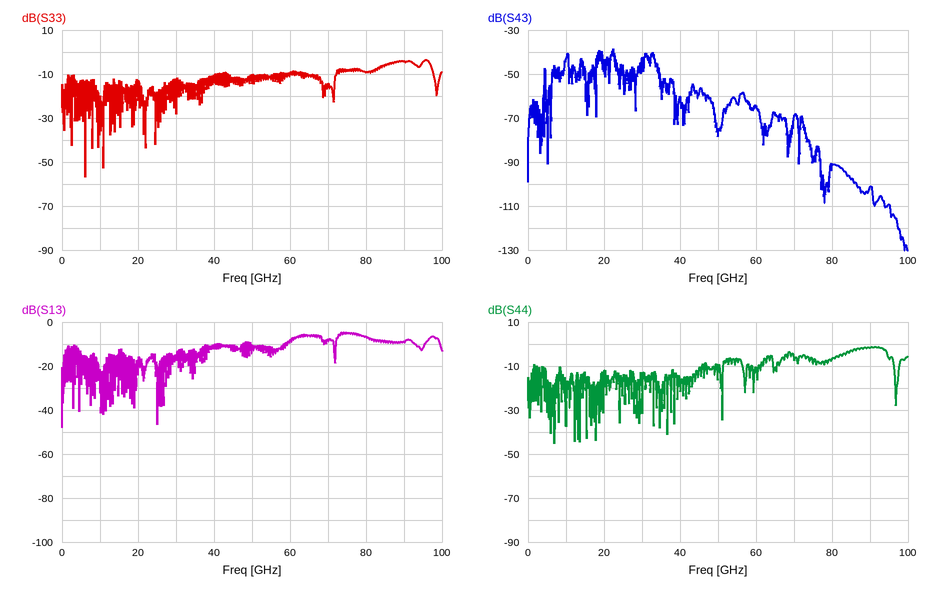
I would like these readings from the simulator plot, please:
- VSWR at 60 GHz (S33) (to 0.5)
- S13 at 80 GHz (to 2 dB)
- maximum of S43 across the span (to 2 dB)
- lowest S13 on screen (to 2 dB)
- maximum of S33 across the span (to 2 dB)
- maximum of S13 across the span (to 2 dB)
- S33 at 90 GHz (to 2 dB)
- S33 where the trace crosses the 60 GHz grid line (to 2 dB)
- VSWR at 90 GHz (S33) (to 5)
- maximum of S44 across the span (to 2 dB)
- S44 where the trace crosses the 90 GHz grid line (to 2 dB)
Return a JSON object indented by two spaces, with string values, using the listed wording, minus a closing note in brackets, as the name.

{
  "VSWR at 60 GHz (S33)": "2.0",
  "S13 at 80 GHz": "-6 dB",
  "maximum of S43 across the span": "-38 dB",
  "lowest S13 on screen": "-48 dB",
  "maximum of S33 across the span": "-4 dB",
  "maximum of S13 across the span": "-4 dB",
  "S33 at 90 GHz": "-4 dB",
  "S33 where the trace crosses the 60 GHz grid line": "-10 dB",
  "VSWR at 90 GHz (S33)": "5",
  "maximum of S44 across the span": "-2 dB",
  "S44 where the trace crosses the 90 GHz grid line": "-2 dB"
}
